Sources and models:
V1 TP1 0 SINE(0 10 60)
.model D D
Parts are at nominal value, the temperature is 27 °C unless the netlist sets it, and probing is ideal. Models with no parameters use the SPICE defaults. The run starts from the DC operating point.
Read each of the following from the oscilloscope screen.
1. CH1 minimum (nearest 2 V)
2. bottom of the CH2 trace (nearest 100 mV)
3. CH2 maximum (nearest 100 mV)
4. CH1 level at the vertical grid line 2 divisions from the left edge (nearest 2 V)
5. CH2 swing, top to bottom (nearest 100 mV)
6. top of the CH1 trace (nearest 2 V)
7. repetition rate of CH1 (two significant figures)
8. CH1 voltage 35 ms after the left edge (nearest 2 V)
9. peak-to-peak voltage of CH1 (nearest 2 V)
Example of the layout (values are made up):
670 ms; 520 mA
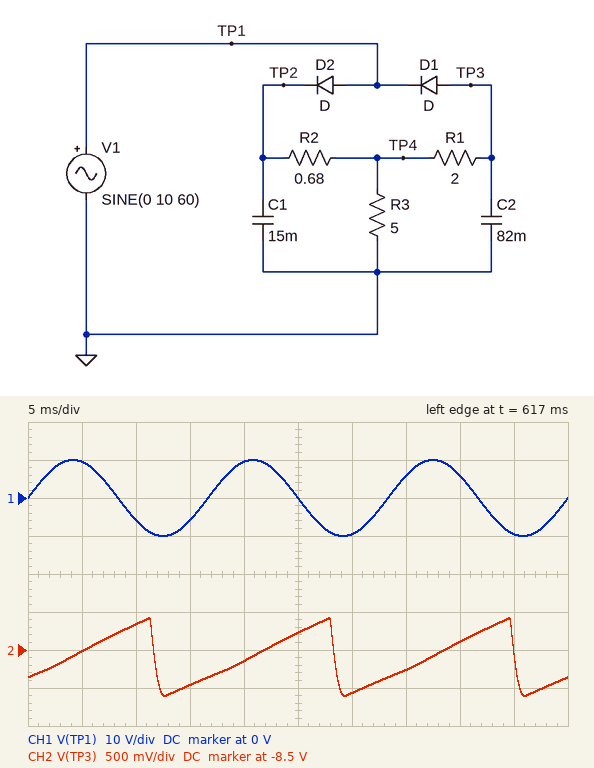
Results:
-10 V; -9.1 V; -8.1 V; -6 V; 1.0 V; 10 V; 60 Hz; 6 V; 20 V
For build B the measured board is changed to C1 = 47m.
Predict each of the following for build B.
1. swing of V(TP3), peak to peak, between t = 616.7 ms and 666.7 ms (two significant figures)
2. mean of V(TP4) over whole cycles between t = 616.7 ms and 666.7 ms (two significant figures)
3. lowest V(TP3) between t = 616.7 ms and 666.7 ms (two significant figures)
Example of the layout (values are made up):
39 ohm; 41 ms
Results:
1.1 V; 3.5 V; -9.1 V
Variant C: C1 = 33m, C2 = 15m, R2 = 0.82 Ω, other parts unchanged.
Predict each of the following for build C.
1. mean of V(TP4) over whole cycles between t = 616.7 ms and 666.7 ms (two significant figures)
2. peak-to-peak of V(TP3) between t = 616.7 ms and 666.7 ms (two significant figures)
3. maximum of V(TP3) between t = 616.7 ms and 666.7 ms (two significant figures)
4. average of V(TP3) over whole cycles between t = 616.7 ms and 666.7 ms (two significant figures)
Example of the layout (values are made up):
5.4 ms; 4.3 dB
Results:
3.2 V; 4.6 V; -4.5 V; -6.9 V
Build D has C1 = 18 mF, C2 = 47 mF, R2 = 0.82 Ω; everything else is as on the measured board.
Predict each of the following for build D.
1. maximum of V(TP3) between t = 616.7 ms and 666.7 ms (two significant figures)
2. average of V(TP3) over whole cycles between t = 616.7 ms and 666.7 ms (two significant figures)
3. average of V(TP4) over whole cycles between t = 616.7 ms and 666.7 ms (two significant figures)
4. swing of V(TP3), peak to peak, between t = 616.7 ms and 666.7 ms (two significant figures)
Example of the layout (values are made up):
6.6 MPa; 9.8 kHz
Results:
-7.4 V; -8.3 V; 2.3 V; 1.7 V
